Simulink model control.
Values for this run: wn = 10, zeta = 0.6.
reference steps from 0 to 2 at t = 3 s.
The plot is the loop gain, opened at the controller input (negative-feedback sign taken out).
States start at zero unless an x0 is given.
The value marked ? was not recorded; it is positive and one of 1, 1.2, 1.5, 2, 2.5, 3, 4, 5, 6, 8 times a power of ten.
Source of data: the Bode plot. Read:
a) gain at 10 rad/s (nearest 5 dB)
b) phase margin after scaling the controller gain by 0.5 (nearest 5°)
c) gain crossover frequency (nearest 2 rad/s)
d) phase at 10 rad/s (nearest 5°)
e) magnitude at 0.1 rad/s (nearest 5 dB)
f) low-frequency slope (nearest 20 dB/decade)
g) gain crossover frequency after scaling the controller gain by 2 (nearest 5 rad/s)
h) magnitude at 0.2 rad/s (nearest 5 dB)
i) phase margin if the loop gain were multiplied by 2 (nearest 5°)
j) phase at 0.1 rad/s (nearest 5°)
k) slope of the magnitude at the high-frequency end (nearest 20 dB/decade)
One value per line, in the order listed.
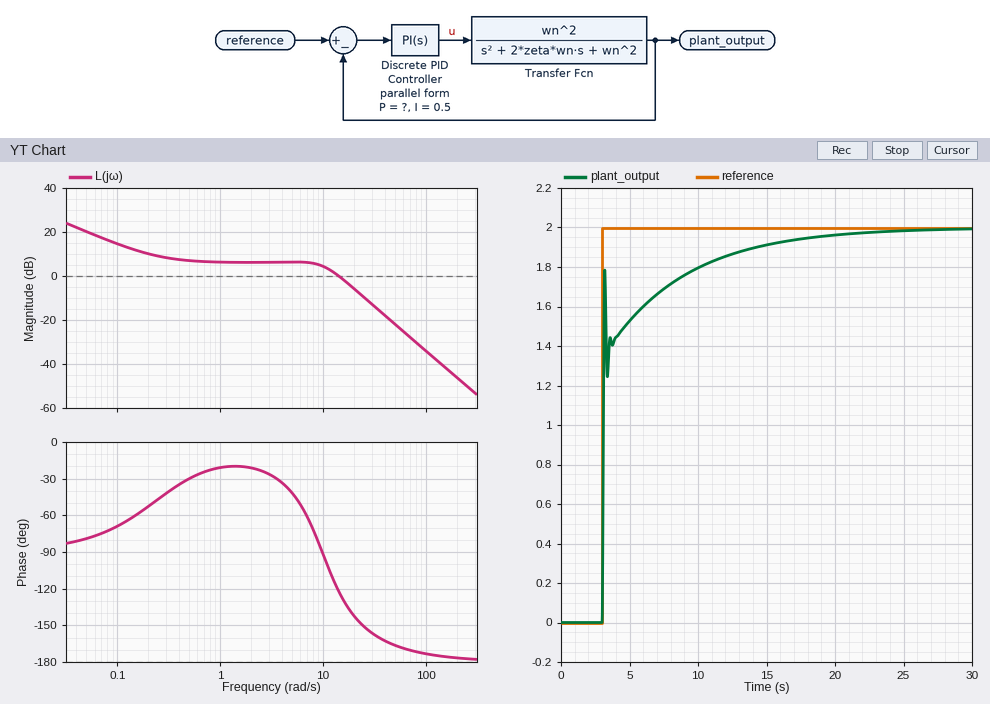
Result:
5 dB
115°
14 rad/s
-90°
15 dB
-20 dB/decade
20 rad/s
10 dB
35°
-70°
-40 dB/decade
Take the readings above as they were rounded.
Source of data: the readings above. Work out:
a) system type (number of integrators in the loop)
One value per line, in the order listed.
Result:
1
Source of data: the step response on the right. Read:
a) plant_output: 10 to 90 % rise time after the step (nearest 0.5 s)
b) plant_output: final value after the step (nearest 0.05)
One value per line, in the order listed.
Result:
7.0 s
2.00
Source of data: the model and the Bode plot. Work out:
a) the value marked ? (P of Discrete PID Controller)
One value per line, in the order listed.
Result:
2
